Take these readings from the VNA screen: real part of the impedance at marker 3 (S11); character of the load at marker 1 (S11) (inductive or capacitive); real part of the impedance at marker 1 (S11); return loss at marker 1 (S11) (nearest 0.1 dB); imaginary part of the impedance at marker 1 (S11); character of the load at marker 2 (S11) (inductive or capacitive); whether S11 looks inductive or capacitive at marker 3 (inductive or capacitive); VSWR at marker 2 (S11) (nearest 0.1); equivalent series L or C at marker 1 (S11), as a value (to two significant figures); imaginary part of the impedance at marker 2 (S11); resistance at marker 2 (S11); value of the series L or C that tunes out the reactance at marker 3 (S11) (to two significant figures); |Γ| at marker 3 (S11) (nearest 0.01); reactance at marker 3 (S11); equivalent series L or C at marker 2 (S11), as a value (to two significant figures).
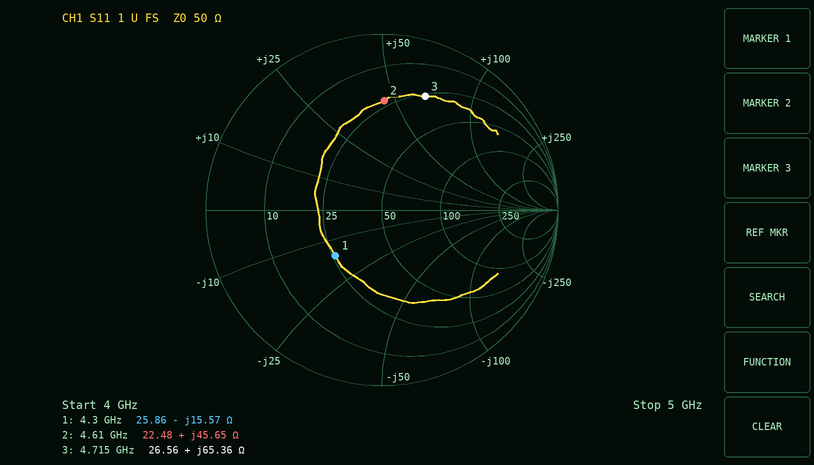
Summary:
26.56 Ω
capacitive
25.86 Ω
8.6 dB
-15.57 Ω
inductive
inductive
4.3
2.4 pF
+45.65 Ω
22.48 Ω
520 fF
0.69
+65.36 Ω
1.6 nH
